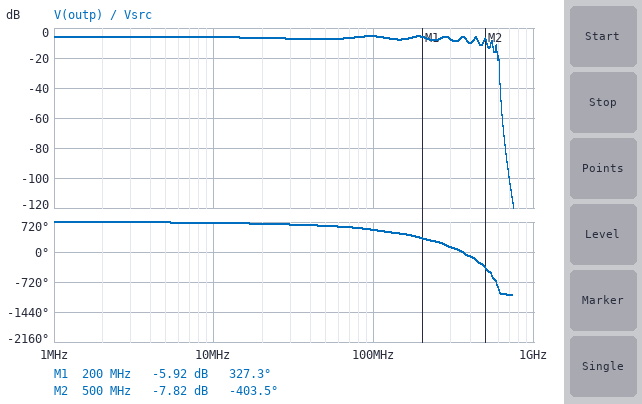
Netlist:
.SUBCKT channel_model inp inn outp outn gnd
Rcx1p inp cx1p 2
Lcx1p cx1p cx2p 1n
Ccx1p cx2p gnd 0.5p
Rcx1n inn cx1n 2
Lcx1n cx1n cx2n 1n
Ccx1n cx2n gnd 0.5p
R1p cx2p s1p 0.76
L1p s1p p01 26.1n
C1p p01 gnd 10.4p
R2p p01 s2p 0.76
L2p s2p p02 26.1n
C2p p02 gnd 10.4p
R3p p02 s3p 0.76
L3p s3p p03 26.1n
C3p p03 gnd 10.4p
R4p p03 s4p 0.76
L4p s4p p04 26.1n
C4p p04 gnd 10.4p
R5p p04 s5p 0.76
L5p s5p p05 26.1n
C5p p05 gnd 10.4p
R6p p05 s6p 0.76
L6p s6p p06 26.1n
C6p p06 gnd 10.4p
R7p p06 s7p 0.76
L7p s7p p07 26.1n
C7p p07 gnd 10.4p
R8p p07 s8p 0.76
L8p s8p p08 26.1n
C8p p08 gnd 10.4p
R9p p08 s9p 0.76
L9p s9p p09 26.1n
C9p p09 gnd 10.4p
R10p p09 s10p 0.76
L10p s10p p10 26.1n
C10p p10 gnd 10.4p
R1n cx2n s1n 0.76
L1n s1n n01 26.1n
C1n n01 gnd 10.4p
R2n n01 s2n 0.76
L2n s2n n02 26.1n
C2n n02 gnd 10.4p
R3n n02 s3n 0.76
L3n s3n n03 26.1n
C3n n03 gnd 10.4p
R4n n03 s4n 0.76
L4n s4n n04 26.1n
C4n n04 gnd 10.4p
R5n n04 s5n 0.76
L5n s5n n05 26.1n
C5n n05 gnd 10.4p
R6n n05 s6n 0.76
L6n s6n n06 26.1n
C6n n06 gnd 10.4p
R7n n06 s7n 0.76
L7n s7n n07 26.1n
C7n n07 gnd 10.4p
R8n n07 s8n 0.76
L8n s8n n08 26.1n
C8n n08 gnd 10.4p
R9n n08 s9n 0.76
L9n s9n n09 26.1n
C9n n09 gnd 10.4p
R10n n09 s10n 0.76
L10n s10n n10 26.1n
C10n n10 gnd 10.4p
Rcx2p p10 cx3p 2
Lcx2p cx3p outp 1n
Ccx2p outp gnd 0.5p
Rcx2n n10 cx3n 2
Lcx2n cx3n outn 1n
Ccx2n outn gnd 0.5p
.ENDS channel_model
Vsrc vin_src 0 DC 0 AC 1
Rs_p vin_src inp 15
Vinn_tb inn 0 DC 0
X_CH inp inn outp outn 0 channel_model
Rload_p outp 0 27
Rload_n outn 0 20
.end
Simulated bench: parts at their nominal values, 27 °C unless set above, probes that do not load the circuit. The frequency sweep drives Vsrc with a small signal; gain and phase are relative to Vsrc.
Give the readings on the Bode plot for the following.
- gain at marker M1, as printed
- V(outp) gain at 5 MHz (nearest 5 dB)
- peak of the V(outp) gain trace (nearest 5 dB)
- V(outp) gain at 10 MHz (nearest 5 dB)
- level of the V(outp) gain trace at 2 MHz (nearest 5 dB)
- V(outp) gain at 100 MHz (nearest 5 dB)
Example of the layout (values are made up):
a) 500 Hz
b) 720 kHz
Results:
a) -5.92 dB
b) -5 dB
c) -5 dB
d) -5 dB
e) -5 dB
f) -5 dB
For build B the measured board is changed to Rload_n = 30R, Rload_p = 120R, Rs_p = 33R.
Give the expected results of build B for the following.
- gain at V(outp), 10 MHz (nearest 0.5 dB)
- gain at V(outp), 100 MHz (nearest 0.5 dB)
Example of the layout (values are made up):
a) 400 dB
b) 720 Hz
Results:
a) -2.5 dB
b) -3.0 dB
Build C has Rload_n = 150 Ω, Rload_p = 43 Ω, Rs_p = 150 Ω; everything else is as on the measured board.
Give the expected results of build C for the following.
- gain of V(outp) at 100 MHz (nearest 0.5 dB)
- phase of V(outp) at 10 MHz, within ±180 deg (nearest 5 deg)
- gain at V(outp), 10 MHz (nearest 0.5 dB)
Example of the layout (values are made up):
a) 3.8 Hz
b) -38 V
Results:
a) -14.0 dB
b) -20 deg
c) -13.5 dB
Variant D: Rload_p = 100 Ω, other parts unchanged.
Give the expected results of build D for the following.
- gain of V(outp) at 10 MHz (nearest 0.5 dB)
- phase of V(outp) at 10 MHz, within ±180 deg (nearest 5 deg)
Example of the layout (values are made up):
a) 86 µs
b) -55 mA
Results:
a) -2.0 dB
b) -15 deg
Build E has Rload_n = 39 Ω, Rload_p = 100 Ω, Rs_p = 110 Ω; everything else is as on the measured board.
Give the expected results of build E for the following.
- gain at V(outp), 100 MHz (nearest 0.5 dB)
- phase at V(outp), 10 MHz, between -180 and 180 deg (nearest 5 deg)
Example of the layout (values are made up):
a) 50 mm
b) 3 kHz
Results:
a) -7.5 dB
b) -25 deg
